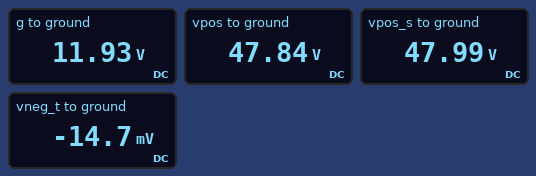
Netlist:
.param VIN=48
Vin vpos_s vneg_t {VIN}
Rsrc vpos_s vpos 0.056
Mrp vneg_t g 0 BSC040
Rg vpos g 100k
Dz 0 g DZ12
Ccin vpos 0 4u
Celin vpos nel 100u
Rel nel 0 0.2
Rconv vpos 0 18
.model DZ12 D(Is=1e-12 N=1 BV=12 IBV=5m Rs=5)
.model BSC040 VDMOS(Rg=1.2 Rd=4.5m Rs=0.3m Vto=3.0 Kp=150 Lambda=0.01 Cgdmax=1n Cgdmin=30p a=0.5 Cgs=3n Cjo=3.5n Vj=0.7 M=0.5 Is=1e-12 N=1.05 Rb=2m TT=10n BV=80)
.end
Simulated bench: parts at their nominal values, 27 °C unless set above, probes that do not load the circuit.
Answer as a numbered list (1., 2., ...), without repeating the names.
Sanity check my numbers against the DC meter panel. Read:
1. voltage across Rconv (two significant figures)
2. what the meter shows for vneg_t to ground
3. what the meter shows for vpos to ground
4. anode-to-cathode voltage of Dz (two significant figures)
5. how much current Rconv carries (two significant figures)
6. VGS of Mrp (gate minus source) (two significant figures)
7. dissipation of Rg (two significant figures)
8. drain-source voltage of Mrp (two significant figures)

1. 48 V
2. -14.7 mV
3. 47.84 V
4. -12 V
5. 2.7 A
6. 12 V
7. 13 mW
8. -15 mV
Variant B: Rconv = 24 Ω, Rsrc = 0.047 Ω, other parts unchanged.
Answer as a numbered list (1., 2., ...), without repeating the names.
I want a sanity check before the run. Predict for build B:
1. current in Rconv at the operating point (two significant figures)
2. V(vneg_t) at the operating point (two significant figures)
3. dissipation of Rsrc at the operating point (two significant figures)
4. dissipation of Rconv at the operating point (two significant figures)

1. 2.0 A
2. -11 mV
3. 190 mW
4. 96 W
